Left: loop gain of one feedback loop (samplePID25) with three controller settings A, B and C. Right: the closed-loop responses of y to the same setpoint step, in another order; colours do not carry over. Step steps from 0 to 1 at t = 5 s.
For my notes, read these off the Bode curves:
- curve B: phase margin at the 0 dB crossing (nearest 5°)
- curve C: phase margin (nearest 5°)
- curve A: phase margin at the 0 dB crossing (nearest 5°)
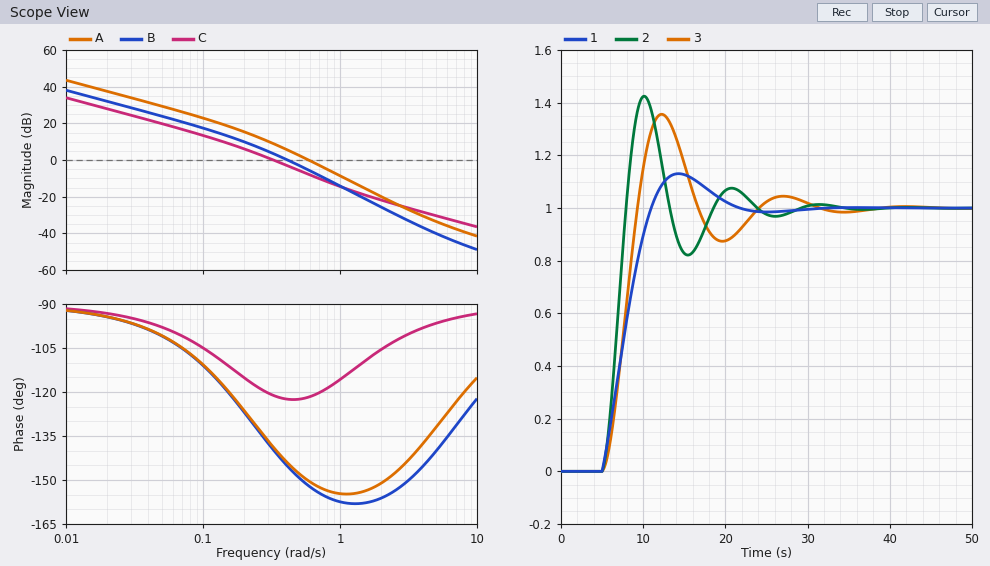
35°
60°
30°
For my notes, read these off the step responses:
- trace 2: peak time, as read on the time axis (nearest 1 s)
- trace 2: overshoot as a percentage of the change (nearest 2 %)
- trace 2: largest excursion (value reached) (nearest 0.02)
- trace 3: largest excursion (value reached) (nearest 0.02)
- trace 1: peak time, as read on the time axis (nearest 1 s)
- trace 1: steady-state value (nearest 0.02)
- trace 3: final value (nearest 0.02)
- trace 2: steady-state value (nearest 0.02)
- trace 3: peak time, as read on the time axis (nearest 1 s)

10 s
42 %
1.42
1.36
14 s
1.00
1.00
1.00
12 s
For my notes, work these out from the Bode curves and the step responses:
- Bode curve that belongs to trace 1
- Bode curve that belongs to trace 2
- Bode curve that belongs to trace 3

C
A
B
